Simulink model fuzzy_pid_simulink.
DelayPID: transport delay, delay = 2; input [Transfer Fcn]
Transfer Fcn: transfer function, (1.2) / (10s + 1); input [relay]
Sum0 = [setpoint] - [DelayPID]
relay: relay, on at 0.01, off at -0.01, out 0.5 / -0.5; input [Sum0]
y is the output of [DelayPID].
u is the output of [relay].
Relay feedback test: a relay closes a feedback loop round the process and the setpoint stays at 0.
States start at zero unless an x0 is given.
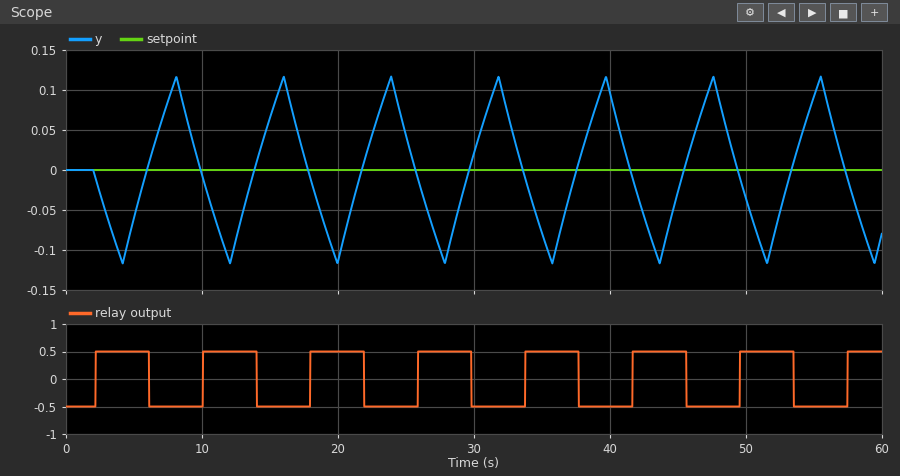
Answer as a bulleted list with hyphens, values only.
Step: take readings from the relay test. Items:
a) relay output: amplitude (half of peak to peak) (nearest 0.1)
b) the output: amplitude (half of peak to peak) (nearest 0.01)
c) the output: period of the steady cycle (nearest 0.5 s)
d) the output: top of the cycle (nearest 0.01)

- 0.5
- 0.12
- 8.0 s
- 0.12
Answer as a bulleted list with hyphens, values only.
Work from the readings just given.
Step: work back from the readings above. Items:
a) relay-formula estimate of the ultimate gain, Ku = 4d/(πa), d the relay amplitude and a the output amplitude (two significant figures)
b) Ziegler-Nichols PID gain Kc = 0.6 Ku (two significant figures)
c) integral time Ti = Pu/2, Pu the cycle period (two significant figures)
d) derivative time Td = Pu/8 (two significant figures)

- 5.3
- 3.2
- 4.0 s
- 1.0 s
